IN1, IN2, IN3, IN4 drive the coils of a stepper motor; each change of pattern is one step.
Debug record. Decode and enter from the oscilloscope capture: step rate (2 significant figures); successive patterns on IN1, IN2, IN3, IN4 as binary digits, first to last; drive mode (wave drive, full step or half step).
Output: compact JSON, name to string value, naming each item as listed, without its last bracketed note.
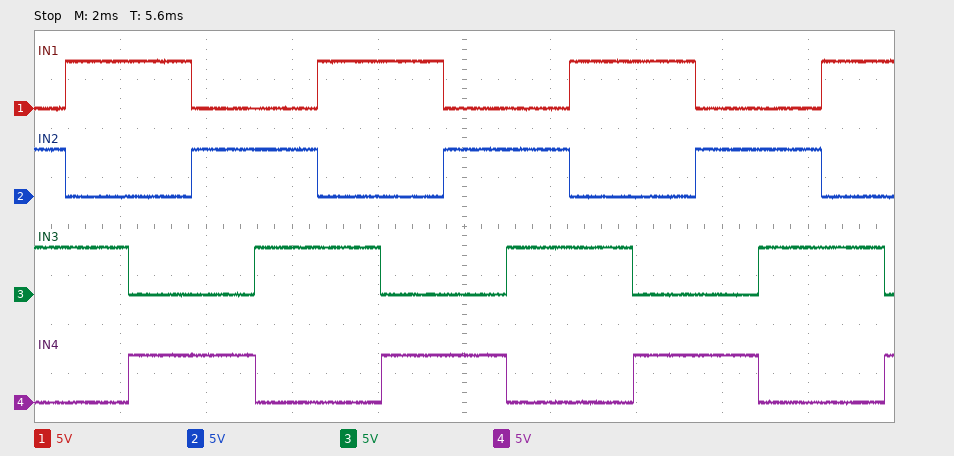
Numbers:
{"step rate": "680 steps/s", "successive patterns on IN1, IN2, IN3, IN4 as binary digits, first to last": "0110 1010 1001 0101 0110 1010 1001 0101 0110 1010 1001 0101 0110 1010 1001", "drive mode": "full step"}
